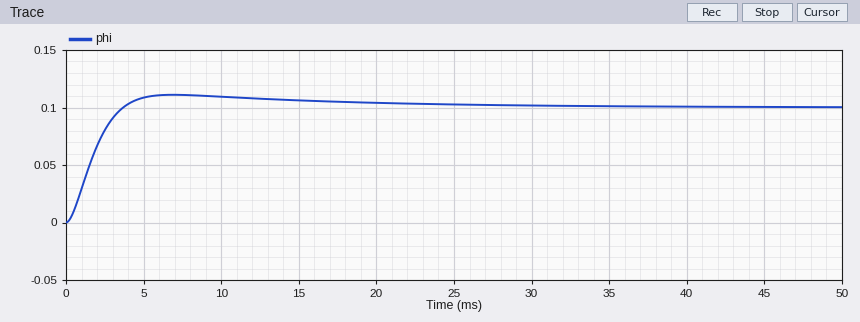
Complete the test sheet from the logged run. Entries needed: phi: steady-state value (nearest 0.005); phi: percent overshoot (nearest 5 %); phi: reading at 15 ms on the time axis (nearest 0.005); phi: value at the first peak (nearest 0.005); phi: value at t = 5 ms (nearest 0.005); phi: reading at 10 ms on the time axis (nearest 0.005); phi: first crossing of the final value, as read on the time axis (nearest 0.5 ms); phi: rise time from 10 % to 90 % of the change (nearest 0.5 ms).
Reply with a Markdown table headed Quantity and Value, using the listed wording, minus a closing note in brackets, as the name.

| Quantity | Value |
|---|---|
| phi: steady-state value | 0.100 |
| phi: percent overshoot | 10 % |
| phi: reading at 15 ms on the time axis | 0.105 |
| phi: value at the first peak | 0.110 |
| phi: value at t = 5 ms | 0.110 |
| phi: reading at 10 ms on the time axis | 0.110 |
| phi: first crossing of the final value, as read on the time axis | 3.5 ms |
| phi: rise time from 10 % to 90 % of the change | 2.5 ms |
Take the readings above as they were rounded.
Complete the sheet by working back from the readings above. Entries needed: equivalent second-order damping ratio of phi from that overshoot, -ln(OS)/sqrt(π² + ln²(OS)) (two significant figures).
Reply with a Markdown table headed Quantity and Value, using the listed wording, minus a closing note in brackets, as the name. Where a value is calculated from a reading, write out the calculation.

| Quantity | Value |
|---|---|
| equivalent second-order damping ratio of phi from that overshoot, -ln(OS)/sqrt(π² + ln²(OS)) | ln(0.1) = -2.303; 2.303 / sqrt(9.870 + 5.302) = 0.59 |
